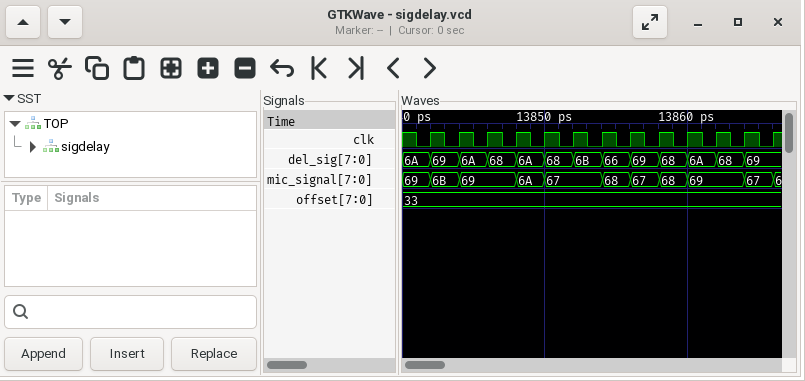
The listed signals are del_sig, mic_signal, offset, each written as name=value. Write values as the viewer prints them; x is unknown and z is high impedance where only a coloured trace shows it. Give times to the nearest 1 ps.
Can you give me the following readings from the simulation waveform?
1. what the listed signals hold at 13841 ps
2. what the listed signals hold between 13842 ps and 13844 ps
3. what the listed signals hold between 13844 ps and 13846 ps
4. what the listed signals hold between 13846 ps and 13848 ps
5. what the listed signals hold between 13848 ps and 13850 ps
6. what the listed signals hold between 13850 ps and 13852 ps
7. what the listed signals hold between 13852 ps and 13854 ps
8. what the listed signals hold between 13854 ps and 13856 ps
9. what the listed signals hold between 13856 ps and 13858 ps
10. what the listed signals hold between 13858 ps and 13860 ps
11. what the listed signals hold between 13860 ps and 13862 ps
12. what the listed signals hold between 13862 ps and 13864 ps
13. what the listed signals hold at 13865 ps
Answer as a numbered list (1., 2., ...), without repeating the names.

1. del_sig=6A, mic_signal=69, offset=33
2. del_sig=69, mic_signal=6B, offset=33
3. del_sig=6A, mic_signal=69, offset=33
4. del_sig=68, mic_signal=69, offset=33
5. del_sig=6A, mic_signal=6A, offset=33
6. del_sig=68, mic_signal=67, offset=33
7. del_sig=6B, mic_signal=67, offset=33
8. del_sig=66, mic_signal=68, offset=33
9. del_sig=69, mic_signal=67, offset=33
10. del_sig=68, mic_signal=68, offset=33
11. del_sig=6A, mic_signal=69, offset=33
12. del_sig=68, mic_signal=69, offset=33
13. del_sig=69, mic_signal=67, offset=33
